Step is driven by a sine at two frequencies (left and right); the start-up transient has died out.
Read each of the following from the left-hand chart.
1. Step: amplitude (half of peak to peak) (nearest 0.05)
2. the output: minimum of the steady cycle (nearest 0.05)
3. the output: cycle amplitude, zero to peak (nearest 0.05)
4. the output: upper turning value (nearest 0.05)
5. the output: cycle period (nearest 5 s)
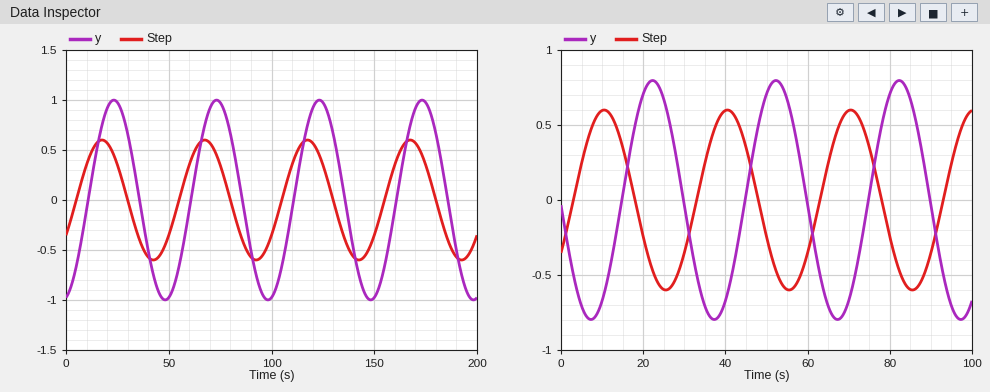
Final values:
0.60
-1.00
1.00
1.00
50 s
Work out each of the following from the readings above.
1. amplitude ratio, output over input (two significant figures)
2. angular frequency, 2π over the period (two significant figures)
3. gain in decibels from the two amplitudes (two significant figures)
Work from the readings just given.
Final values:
1.7
0.13 rad/s
4.4 dB
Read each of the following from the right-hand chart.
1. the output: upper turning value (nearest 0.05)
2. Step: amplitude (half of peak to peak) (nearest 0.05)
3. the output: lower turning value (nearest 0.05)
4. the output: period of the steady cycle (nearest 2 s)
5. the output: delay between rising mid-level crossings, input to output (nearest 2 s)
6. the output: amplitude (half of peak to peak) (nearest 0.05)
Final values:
0.80
0.60
-0.80
30 s
12 s
0.80
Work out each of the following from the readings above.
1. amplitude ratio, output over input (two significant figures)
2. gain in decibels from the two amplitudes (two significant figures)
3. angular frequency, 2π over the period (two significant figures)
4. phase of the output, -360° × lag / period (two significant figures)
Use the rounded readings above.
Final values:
1.3
2.5 dB
0.21 rad/s
-140°
